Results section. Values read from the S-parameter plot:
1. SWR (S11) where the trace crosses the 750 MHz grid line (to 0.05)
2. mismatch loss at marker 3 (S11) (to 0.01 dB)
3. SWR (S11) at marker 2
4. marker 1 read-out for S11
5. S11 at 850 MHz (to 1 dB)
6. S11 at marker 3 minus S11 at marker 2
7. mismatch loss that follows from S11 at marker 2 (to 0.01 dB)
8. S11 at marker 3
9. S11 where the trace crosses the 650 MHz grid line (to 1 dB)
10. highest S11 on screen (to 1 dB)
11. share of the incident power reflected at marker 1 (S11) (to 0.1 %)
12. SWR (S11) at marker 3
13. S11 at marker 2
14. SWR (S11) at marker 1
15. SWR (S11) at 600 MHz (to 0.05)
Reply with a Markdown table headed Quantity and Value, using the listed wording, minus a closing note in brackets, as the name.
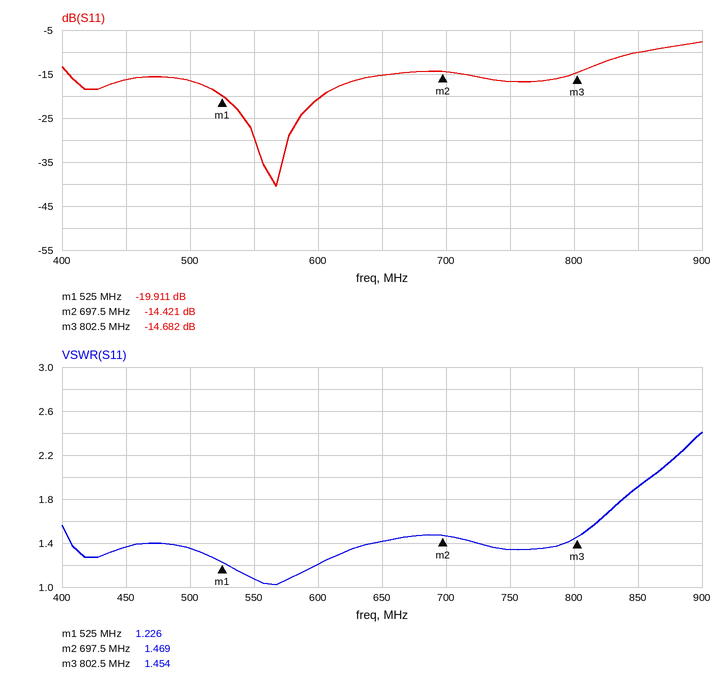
| Quantity | Value |
|---|---|
| SWR (S11) where the trace crosses the 750 MHz grid line | 1.35 |
| mismatch loss at marker 3 (S11) | 0.15 dB |
| SWR (S11) at marker 2 | 1.469 |
| marker 1 read-out for S11 | -19.911 dB |
| S11 at 850 MHz | -10 dB |
| S11 at marker 3 minus S11 at marker 2 | -0.261 dB |
| mismatch loss that follows from S11 at marker 2 | 0.16 dB |
| S11 at marker 3 | -14.682 dB |
| S11 where the trace crosses the 650 MHz grid line | -15 dB |
| highest S11 on screen | -8 dB |
| share of the incident power reflected at marker 1 (S11) | 1.0 % |
| SWR (S11) at marker 3 | 1.454 |
| S11 at marker 2 | -14.421 dB |
| SWR (S11) at marker 1 | 1.226 |
| SWR (S11) at 600 MHz | 1.20 |
